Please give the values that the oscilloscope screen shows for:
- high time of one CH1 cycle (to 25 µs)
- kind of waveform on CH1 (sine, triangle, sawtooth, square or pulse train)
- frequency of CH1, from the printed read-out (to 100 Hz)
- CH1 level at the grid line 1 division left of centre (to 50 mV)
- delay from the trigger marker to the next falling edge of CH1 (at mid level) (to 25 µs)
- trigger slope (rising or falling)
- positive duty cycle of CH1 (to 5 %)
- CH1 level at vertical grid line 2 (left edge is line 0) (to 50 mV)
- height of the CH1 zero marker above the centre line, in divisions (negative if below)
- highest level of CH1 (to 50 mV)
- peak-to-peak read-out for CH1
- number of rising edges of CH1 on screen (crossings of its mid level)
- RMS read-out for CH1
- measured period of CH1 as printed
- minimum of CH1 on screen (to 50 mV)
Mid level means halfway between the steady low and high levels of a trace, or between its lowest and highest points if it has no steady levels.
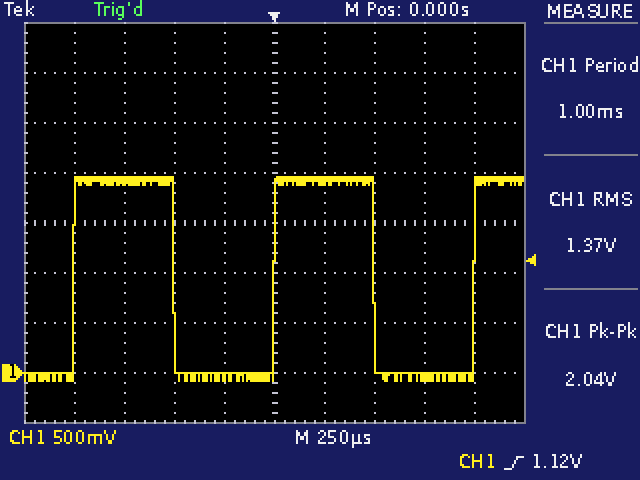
500 µs
square
1.0 kHz
-50 mV
500 µs
rising
50 %
1.90 V
-3.0 div
1.95 V
2.04 V
3
1.37 V
1.00 ms
-100 mV
